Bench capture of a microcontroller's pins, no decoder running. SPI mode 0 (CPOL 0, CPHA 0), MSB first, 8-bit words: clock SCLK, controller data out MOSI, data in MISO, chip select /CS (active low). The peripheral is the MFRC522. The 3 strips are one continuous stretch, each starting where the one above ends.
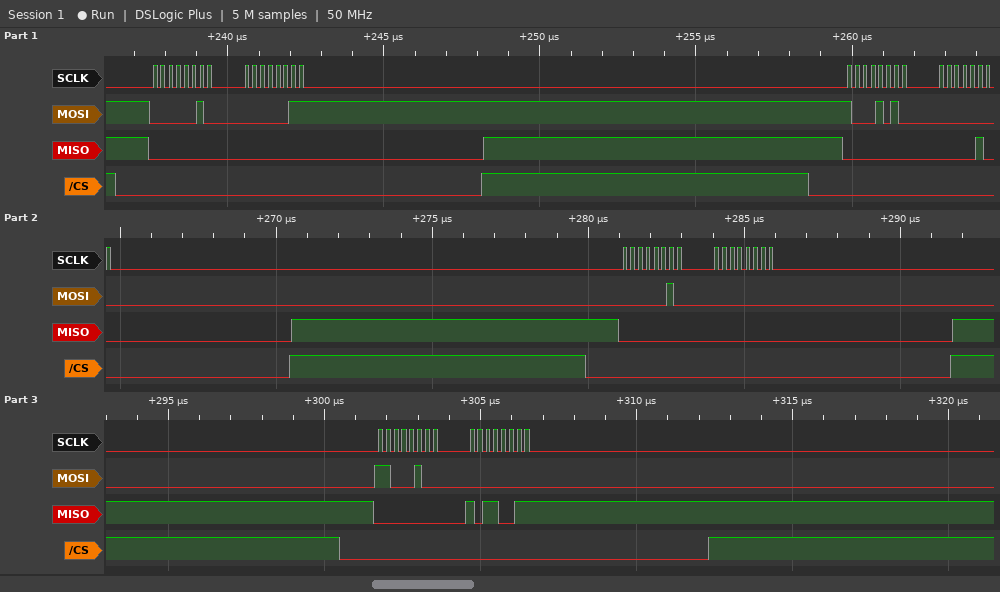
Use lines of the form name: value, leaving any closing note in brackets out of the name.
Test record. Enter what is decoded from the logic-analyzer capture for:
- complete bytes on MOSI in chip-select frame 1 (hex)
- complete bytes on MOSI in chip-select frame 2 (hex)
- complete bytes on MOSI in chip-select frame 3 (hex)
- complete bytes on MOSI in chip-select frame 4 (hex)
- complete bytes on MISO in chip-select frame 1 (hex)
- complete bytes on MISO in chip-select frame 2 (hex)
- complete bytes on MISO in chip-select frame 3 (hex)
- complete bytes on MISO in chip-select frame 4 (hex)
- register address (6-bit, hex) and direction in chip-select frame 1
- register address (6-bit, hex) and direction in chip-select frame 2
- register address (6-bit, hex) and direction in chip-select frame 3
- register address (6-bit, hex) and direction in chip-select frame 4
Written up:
complete bytes on MOSI in chip-select frame 1: 02 03
complete bytes on MOSI in chip-select frame 2: 8A 00
complete bytes on MOSI in chip-select frame 3: 02 00
complete bytes on MOSI in chip-select frame 4: C4 00
complete bytes on MISO in chip-select frame 1: 00 00
complete bytes on MISO in chip-select frame 2: 00 04
complete bytes on MISO in chip-select frame 3: 00 00
complete bytes on MISO in chip-select frame 4: 00 B3
register address (6-bit, hex) and direction in chip-select frame 1: 0x01 write
register address (6-bit, hex) and direction in chip-select frame 2: 0x05 read
register address (6-bit, hex) and direction in chip-select frame 3: 0x01 write
register address (6-bit, hex) and direction in chip-select frame 4: 0x22 read
